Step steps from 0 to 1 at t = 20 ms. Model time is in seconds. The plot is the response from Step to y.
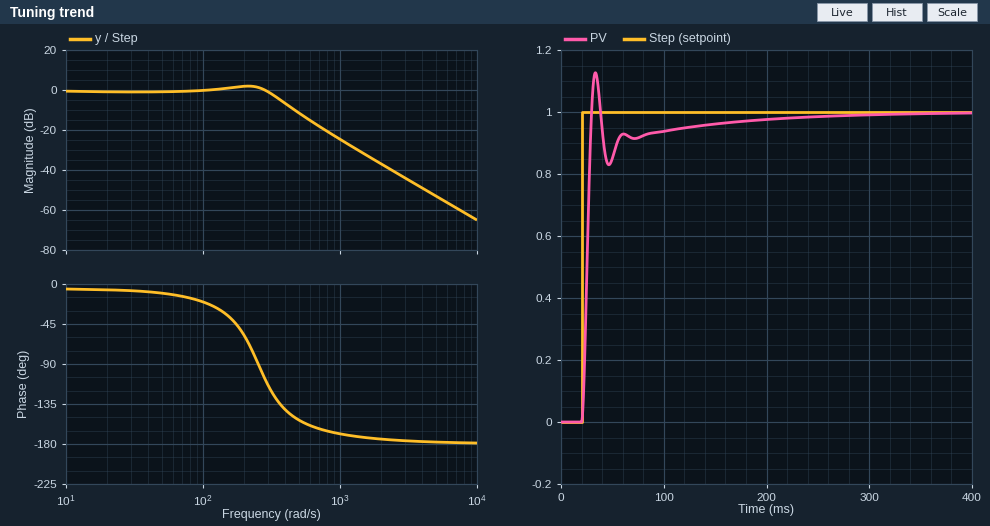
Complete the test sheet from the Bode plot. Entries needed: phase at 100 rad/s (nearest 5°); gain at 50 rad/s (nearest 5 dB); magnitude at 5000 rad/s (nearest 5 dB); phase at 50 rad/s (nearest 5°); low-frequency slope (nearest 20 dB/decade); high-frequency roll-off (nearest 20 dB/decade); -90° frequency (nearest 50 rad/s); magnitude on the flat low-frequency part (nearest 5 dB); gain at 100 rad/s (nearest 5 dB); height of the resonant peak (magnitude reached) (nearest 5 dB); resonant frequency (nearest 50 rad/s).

-20°
0 dB
-55 dB
-10°
0 dB/decade
-40 dB/decade
250 rad/s
0 dB
0 dB
0 dB
200 rad/s
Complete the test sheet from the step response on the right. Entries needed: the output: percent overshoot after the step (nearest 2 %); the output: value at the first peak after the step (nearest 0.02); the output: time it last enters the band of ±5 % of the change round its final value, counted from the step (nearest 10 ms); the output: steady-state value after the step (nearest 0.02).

12 %
1.12
100 ms
1.00
